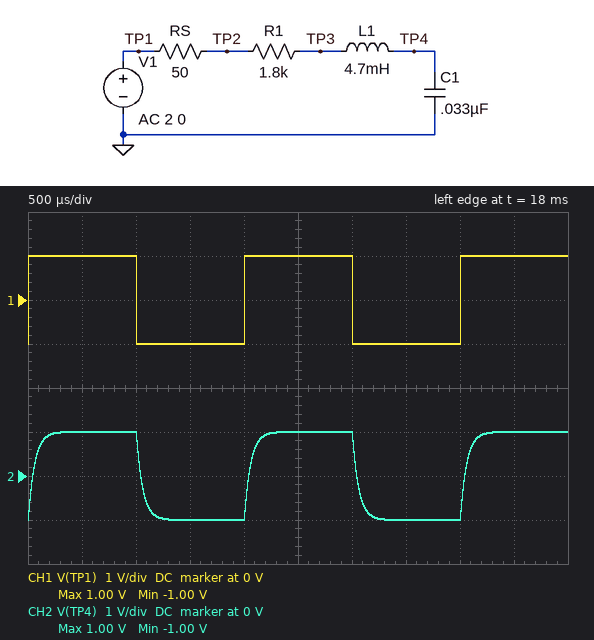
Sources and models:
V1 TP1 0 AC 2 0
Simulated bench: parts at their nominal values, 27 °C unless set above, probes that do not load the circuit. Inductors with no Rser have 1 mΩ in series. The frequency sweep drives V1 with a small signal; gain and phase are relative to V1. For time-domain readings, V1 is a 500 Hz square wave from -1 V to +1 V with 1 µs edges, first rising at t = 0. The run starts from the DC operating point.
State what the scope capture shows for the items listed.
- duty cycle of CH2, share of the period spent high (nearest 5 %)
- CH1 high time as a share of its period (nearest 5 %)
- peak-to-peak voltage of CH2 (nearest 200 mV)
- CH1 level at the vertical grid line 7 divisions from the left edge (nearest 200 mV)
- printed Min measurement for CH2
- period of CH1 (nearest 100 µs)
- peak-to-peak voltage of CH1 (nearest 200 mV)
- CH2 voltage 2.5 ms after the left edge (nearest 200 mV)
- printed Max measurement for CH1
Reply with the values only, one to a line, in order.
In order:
50 %
50 %
2.0 V
-1.0 V
-1.00 V
2.0 ms
2.0 V
1.0 V
1.00 V
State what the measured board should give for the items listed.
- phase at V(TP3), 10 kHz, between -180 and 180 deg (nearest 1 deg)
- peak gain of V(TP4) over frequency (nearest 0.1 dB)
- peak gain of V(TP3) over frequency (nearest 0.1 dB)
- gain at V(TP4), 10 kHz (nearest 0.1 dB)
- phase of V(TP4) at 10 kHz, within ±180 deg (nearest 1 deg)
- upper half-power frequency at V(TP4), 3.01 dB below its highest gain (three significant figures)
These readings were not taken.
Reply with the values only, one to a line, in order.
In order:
-84 deg
0 dB
0 dB
-11.7 dB
-84 deg
2.72 kHz
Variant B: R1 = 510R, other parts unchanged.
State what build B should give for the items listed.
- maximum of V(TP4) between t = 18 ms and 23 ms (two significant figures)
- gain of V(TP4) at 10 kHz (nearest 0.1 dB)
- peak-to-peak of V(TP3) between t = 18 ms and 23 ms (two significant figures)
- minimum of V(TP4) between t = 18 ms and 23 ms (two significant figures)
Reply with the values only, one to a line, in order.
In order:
1.1 V
-1.8 dB
2.1 V
-1.1 V
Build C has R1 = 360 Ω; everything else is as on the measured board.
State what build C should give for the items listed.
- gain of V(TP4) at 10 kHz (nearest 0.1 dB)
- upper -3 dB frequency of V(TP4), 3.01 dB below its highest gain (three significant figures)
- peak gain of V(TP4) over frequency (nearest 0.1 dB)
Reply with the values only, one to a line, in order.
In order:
0.6 dB
14.7 kHz
0.8 dB
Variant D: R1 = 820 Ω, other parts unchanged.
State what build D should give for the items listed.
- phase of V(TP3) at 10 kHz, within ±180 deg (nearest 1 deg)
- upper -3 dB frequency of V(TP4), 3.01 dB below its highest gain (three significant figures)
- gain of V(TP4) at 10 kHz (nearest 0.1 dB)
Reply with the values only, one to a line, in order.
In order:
-78 deg
6.74 kHz
-5.3 dB
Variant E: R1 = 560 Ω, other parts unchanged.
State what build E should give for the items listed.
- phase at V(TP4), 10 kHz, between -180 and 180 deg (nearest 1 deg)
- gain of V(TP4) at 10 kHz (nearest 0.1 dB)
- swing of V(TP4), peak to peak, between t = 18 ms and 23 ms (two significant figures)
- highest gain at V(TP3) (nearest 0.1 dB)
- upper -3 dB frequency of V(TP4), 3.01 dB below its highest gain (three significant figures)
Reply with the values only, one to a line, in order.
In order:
-73 deg
-2.4 dB
2.1 V
0 dB
11.0 kHz
